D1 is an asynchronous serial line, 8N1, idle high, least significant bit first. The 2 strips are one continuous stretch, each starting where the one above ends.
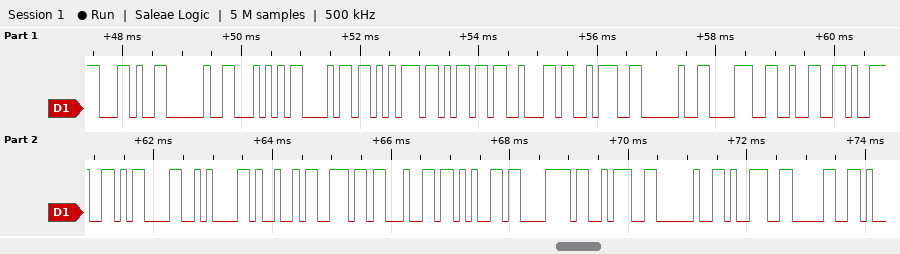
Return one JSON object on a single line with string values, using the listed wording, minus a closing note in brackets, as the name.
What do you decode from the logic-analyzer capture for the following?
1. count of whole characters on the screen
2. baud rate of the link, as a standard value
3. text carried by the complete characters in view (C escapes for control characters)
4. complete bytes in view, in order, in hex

{"count of whole characters on the screen": "23", "baud rate of the link, as a standard value": "9600 baud", "text carried by the complete characters in view": "\", Thumb: 829\\r\\nIndex: 90\"", "complete bytes in view, in order, in hex": "2C 20 54 68 75 6D 62 3A 20 38 32 39 0D 0A 49 6E 64 65 78 3A 20 39 30"}
